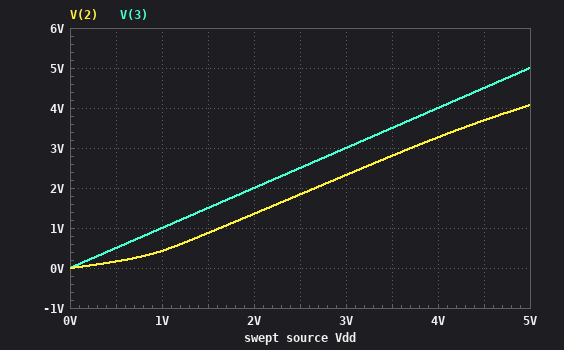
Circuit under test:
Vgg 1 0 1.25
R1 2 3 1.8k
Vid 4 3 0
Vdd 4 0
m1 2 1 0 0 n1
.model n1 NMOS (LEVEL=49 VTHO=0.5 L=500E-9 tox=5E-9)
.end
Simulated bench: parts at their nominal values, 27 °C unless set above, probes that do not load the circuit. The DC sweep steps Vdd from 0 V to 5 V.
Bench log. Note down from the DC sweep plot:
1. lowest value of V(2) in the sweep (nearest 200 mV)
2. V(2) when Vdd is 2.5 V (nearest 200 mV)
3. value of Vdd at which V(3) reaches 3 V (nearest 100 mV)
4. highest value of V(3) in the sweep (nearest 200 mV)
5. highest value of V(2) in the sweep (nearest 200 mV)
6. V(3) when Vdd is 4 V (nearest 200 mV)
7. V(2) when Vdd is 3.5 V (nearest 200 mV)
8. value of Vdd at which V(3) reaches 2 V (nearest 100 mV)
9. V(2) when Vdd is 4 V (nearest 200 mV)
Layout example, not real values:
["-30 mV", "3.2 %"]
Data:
["0 V", "1.8 V", "3.0 V", "5.0 V", "4.0 V", "4.0 V", "2.8 V", "2.0 V", "3.2 V"]
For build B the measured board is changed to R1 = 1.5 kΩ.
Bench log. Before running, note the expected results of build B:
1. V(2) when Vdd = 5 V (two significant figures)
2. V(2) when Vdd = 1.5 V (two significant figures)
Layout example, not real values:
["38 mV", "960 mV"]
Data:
["4.2 V", "970 mV"]
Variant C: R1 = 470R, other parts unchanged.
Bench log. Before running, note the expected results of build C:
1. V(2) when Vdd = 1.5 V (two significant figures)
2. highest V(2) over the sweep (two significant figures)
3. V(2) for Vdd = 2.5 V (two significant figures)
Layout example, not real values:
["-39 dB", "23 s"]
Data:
["1.3 V", "4.7 V", "2.3 V"]
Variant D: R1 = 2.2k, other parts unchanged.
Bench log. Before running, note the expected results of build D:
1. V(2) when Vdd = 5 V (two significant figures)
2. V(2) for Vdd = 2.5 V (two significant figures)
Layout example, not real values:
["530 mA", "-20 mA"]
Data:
["3.9 V", "1.7 V"]
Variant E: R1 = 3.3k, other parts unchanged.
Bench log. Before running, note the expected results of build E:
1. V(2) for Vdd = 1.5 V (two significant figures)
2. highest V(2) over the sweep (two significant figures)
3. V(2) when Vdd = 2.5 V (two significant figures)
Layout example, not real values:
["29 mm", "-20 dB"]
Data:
["440 mV", "3.6 V", "1.3 V"]
